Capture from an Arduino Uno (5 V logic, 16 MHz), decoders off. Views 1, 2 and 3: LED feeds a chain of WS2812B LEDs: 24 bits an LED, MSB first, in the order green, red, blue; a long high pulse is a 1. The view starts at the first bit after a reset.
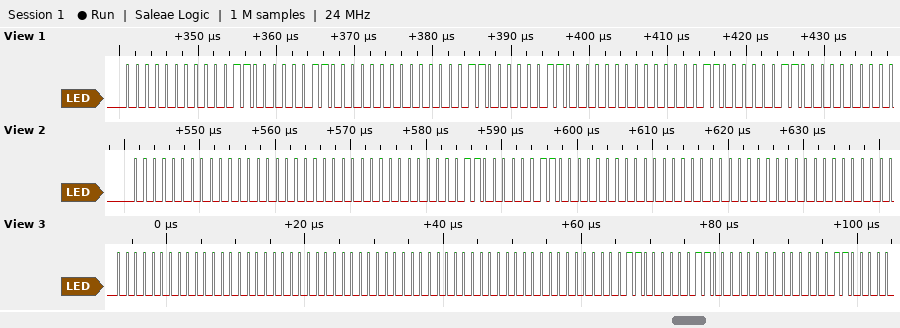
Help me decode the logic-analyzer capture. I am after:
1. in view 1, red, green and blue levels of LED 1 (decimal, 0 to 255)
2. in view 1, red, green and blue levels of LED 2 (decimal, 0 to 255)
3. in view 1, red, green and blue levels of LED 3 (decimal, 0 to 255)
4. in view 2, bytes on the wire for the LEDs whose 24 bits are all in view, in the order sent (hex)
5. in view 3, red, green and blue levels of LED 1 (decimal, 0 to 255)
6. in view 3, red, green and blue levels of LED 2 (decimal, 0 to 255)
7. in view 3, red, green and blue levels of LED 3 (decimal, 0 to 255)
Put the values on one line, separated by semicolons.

24, 0, 24; 24, 0, 24; 24, 0, 24; 00 00 00 00 18 18 00 00 00; 0, 0, 0; 0, 0, 0; 24, 0, 24
